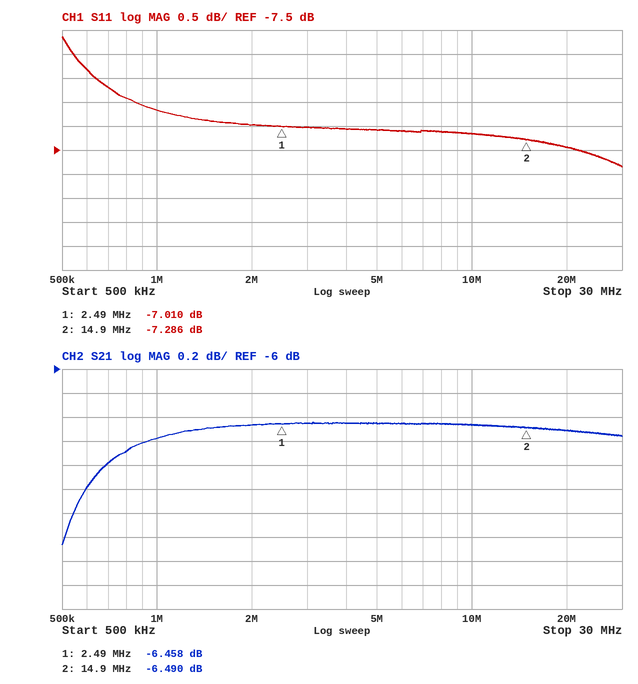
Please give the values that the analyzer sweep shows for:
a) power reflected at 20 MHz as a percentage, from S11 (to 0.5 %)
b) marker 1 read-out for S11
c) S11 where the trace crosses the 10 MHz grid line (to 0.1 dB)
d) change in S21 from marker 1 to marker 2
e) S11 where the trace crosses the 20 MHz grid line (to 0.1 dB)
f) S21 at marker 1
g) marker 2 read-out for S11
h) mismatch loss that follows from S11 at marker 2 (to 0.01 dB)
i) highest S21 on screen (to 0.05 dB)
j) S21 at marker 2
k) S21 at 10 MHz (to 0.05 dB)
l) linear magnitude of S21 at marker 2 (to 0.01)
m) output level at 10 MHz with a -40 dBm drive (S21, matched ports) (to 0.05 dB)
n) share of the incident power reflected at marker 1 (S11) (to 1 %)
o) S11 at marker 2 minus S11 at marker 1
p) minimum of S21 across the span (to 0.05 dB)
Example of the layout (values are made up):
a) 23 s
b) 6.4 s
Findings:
a) 18.0 %
b) -7.010 dB
c) -7.2 dB
d) -0.032 dB
e) -7.4 dB
f) -6.458 dB
g) -7.286 dB
h) 0.90 dB
i) -6.45 dB
j) -6.490 dB
k) -6.45 dB
l) 0.47
m) -46.45 dBm
n) 20 %
o) -0.276 dB
p) -7.45 dB
